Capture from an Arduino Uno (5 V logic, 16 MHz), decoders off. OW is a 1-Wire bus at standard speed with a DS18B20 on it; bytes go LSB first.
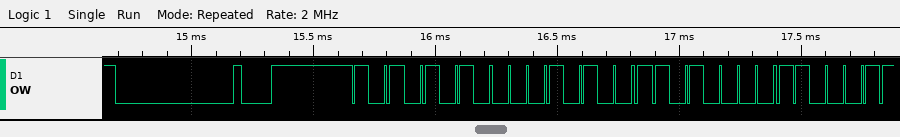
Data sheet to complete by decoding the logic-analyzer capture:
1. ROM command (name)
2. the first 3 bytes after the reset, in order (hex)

Match ROM
55 28 0B
